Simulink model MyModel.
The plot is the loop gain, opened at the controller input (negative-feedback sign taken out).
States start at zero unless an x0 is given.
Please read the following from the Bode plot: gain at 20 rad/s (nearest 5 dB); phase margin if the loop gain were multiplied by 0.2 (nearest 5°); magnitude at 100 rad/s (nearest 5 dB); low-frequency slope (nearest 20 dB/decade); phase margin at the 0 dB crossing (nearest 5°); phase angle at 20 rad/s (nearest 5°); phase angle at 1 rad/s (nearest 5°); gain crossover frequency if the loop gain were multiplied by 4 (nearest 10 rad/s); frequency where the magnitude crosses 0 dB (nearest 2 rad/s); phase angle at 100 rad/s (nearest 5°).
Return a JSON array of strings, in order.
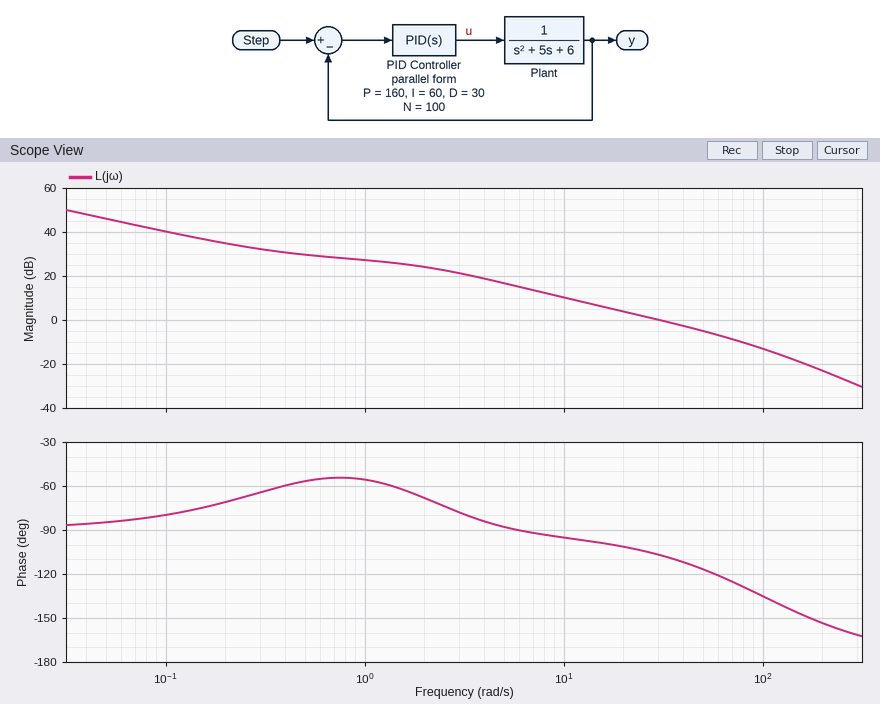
["5 dB", "90°", "-15 dB", "-20 dB/decade", "75°", "-100°", "-55°", "90 rad/s", "30 rad/s", "-135°"]
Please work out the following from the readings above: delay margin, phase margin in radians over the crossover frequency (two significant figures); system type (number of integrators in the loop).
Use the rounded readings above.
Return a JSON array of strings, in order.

["0.044 s", "1"]
